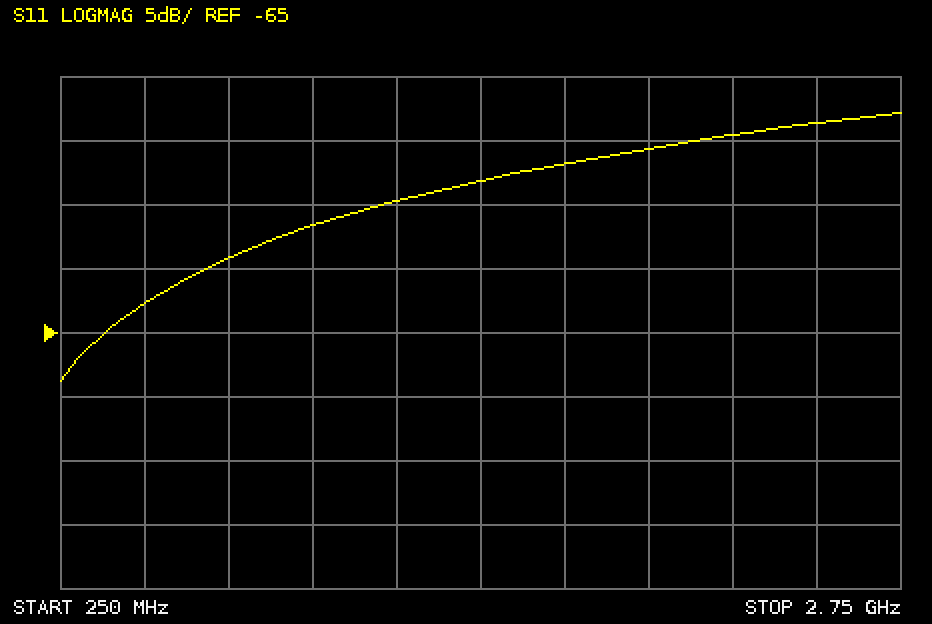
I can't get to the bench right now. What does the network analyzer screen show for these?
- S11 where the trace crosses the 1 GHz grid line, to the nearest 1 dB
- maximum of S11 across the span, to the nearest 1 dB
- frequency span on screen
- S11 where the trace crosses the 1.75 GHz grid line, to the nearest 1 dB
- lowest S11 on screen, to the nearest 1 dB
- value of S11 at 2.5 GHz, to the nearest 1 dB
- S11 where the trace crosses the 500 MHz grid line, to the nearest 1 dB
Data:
-57 dB
-48 dB
2.5 GHz
-52 dB
-69 dB
-49 dB
-63 dB
